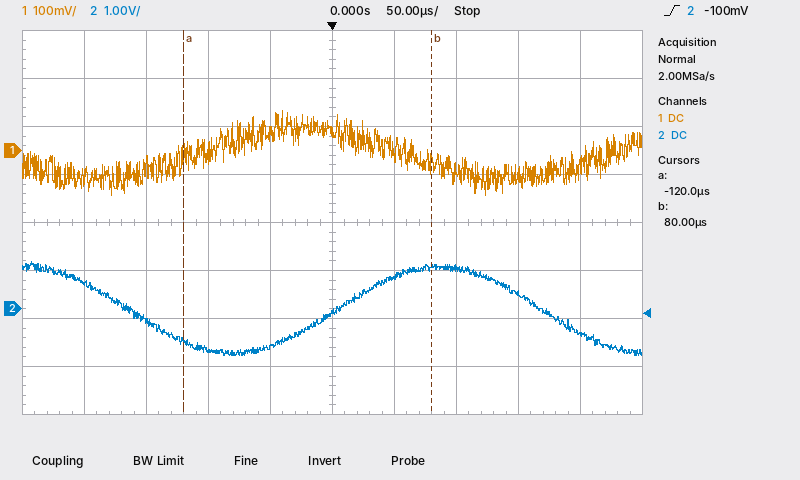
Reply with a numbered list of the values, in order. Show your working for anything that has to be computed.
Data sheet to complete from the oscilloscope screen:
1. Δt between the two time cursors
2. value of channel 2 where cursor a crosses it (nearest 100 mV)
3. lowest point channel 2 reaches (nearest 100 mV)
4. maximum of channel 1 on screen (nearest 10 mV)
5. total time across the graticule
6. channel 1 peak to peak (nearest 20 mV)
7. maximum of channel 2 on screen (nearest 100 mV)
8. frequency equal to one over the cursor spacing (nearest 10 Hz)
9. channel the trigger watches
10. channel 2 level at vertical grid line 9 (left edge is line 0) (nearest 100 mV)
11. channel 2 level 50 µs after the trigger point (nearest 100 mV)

1. 80 µs − (-120 µs) = 200 µs
2. -700 mV
3. -1.0 V
4. 80 mV
5. 500 µs
6. 180 mV
7. 1.0 V
8. 1 / 200 µs ≈ 5.00 kHz
9. channel 2
10. -500 mV
11. 700 mV
